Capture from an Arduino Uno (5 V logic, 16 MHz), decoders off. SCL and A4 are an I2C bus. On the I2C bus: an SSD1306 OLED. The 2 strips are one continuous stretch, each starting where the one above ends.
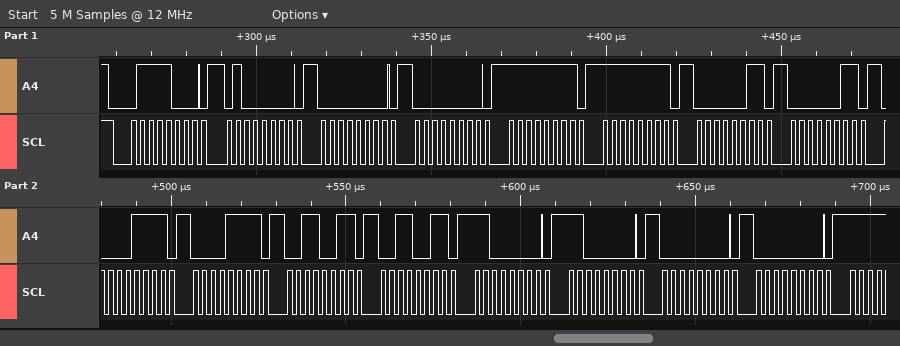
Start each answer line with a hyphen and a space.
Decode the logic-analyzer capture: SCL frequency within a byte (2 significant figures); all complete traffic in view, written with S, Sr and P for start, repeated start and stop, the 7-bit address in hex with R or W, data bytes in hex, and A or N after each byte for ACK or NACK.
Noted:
- 400 kHz
- S 3CW A 40 A 00 A 00 A FF A FF A 03 A 03 A 0F A 0F A 33 A 33 A C0 A C0 A 00 A 00 A
